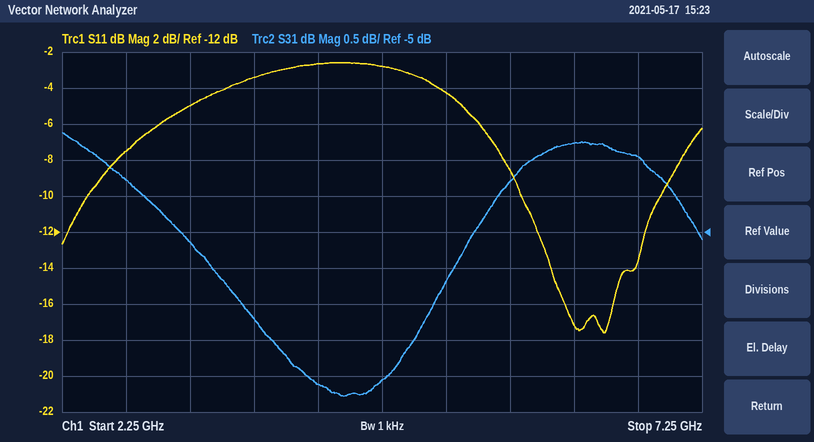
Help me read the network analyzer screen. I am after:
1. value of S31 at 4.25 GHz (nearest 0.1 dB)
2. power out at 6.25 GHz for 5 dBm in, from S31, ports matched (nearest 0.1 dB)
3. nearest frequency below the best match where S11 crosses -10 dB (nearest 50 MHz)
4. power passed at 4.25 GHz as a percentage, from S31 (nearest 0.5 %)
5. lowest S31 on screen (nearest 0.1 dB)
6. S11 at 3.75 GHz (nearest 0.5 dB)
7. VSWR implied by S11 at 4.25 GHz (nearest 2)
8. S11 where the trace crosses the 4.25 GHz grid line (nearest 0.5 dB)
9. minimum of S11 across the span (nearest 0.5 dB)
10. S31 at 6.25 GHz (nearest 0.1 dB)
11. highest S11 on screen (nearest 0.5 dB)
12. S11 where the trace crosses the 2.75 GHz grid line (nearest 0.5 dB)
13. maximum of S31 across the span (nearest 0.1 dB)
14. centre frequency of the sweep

-7.1 dB
1.2 dBm
5.85 GHz
19.5 %
-7.3 dB
-3.5 dB
6
-2.5 dB
-17.5 dB
-3.8 dB
-2.5 dB
-7.5 dB
-3.6 dB
4.75 GHz
